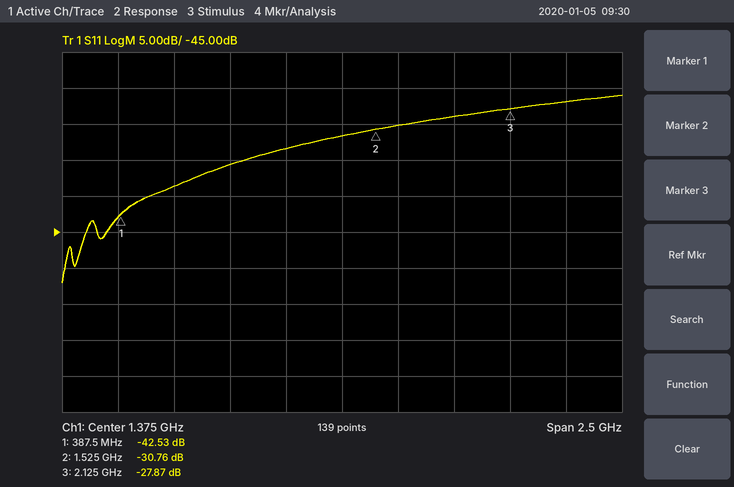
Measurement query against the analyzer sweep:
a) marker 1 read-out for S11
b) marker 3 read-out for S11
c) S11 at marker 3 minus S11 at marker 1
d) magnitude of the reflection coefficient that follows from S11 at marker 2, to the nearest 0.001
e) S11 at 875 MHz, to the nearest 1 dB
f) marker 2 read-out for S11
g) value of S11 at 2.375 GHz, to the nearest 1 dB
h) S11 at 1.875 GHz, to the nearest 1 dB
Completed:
-42.53 dB
-27.87 dB
14.66 dB
0.029
-36 dB
-30.76 dB
-27 dB
-29 dB
